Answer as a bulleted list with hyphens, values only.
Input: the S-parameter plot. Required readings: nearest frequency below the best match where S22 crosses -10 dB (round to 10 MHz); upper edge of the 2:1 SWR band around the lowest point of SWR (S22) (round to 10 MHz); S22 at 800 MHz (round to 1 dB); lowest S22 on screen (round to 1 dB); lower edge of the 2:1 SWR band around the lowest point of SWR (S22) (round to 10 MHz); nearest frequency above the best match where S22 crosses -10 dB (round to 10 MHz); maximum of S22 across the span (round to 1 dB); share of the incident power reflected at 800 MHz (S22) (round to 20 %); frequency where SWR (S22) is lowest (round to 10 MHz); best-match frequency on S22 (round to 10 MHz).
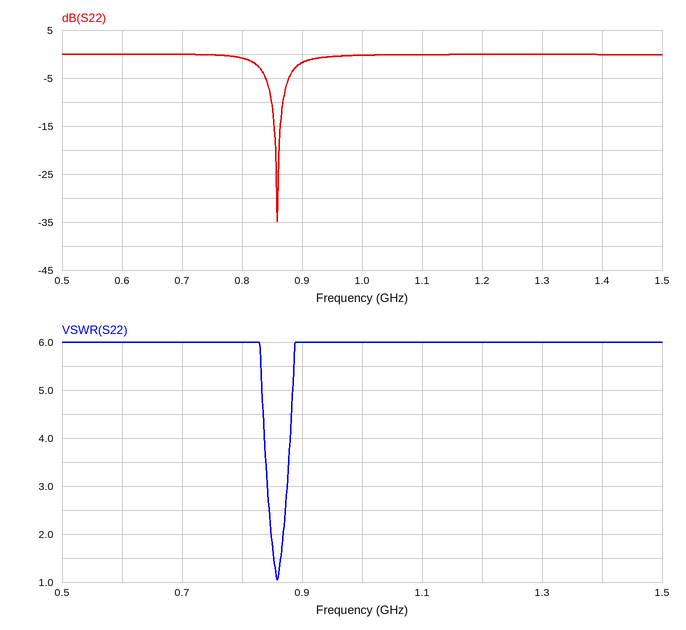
- 850 MHz
- 870 MHz
- -1 dB
- -35 dB
- 850 MHz
- 870 MHz
- 0 dB
- 80 %
- 860 MHz
- 860 MHz
